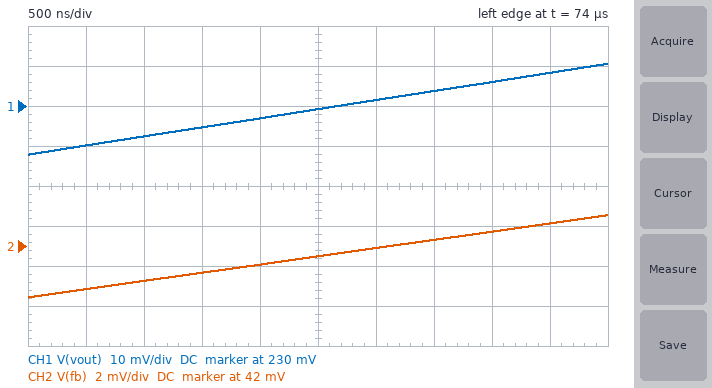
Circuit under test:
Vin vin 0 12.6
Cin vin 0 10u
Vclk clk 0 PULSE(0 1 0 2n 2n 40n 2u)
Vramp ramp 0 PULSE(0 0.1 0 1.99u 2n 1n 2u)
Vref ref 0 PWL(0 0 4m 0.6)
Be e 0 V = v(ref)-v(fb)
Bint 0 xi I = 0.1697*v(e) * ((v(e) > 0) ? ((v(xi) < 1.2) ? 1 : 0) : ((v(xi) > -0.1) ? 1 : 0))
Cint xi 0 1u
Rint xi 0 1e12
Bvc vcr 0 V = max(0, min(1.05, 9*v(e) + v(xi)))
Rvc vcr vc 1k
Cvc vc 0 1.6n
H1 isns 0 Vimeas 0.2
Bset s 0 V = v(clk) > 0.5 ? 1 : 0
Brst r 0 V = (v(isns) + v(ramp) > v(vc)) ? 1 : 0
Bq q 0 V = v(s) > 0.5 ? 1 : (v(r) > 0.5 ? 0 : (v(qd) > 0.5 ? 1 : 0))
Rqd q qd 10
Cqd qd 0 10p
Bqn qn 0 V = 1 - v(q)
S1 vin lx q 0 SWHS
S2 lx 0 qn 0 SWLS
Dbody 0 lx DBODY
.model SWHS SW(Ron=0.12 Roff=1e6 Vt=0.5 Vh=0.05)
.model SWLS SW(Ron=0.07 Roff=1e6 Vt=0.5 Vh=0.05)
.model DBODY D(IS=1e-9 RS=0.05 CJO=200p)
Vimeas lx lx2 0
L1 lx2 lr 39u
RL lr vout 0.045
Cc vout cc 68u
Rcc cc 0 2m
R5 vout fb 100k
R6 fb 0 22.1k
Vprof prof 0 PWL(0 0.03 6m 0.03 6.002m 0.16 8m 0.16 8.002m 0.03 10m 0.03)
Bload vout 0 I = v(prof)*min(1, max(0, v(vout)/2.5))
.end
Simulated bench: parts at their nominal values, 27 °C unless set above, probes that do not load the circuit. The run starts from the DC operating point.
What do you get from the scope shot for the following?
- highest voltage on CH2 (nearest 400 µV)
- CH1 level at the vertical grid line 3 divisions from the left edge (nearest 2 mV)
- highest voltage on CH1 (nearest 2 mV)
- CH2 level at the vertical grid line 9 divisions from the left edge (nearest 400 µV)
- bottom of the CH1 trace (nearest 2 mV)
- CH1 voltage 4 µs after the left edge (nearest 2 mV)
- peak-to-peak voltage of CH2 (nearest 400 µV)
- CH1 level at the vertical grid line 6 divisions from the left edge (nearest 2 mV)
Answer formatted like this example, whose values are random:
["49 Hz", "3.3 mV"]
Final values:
["43.6 mV", "224 mV", "240 mV", "43.2 mV", "218 mV", "236 mV", "4.0 mV", "232 mV"]
